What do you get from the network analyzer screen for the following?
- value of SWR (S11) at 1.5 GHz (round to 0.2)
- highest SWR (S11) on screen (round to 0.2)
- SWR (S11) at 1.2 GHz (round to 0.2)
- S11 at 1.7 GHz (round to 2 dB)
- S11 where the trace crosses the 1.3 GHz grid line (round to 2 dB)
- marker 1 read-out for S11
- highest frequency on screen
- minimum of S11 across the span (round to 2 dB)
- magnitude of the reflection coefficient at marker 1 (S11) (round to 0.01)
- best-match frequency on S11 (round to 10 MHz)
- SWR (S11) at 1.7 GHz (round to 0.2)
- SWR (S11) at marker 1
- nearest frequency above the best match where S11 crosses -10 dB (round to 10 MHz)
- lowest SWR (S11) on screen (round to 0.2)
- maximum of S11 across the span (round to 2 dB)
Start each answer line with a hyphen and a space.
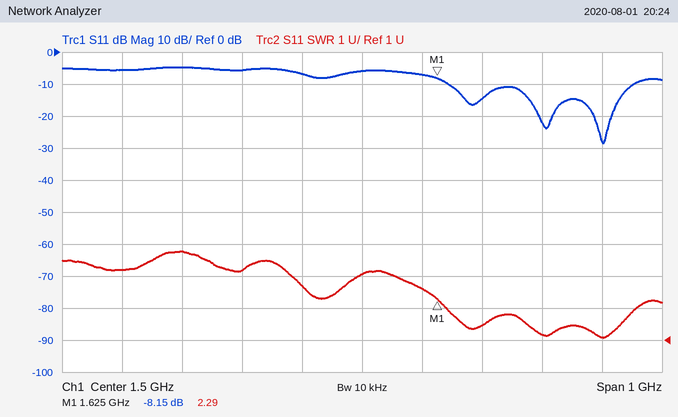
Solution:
- 3.0
- 3.8
- 3.8
- -14 dB
- -6 dB
- -8.15 dB
- 2 GHz
- -28 dB
- 0.39
- 1.90 GHz
- 1.4
- 2.29
- 1.95 GHz
- 1.0
- -4 dB
